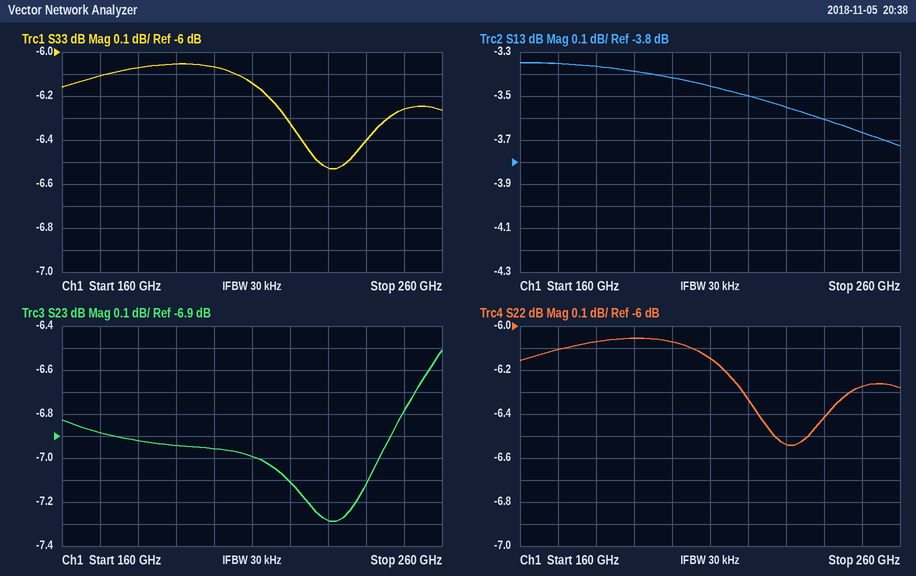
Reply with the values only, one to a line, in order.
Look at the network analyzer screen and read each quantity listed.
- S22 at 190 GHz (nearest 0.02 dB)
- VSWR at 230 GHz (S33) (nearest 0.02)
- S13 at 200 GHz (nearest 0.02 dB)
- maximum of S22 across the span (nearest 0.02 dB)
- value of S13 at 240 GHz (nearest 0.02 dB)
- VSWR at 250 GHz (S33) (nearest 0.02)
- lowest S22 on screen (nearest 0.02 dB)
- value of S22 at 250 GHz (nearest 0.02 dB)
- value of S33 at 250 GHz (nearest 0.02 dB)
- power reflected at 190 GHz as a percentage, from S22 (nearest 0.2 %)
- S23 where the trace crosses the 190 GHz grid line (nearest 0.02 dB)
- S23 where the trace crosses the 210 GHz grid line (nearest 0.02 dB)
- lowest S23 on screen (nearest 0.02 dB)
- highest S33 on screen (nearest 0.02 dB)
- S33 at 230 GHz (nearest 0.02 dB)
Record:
-6.06 dB
2.78
-3.42 dB
-6.06 dB
-3.60 dB
2.90
-6.54 dB
-6.28 dB
-6.26 dB
24.8 %
-6.94 dB
-7.00 dB
-7.28 dB
-6.06 dB
-6.52 dB
